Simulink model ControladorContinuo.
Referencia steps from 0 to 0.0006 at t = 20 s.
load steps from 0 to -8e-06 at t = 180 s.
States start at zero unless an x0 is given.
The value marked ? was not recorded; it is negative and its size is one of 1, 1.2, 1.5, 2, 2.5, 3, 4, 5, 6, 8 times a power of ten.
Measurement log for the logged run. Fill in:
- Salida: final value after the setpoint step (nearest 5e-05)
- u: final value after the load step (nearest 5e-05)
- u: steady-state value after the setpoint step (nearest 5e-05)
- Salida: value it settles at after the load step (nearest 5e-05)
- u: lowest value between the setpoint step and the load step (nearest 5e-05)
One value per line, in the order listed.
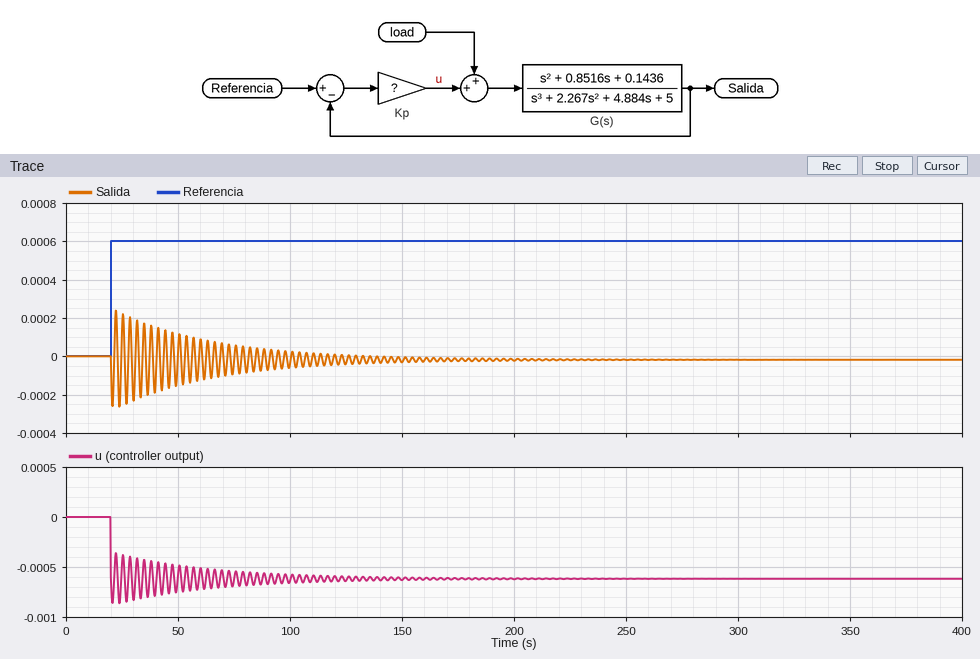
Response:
0.00000
-0.00060
-0.00060
0.00000
-0.00085
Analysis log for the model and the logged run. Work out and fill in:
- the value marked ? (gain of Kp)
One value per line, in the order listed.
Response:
-1
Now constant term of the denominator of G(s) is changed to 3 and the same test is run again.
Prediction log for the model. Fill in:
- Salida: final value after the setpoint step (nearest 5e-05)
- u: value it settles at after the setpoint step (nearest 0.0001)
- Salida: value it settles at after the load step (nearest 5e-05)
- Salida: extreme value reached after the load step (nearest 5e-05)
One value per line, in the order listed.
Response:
-0.00005
-0.0006
-0.00005
-0.00005
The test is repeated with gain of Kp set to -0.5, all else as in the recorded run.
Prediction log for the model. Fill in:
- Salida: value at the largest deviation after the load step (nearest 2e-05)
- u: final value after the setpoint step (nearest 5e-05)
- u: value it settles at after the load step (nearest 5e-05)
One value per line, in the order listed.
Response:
-0.00002
-0.00030
-0.00030
